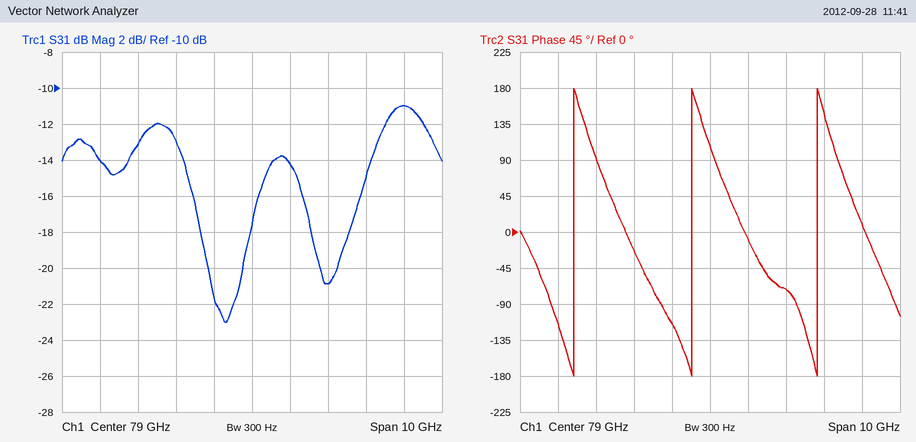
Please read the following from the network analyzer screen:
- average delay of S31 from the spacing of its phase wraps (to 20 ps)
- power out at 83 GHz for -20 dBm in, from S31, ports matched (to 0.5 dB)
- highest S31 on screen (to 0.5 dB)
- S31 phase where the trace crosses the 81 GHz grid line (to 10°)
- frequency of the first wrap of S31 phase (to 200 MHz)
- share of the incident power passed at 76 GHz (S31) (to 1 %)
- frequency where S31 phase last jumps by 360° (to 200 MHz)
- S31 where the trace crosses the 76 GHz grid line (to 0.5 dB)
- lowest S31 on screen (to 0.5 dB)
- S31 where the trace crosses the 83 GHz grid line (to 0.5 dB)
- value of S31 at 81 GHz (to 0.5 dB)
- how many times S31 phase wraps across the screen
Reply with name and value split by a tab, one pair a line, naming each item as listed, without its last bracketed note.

average delay of S31 from the spacing of its phase wraps	320 ps
power out at 83 GHz for -20 dBm in, from S31, ports matched	-31.0 dBm
highest S31 on screen	-11.0 dB
S31 phase where the trace crosses the 81 GHz grid line	-70°
frequency of the first wrap of S31 phase	75.4 GHz
share of the incident power passed at 76 GHz (S31)	5 %
frequency where S31 phase last jumps by 360°	81.8 GHz
S31 where the trace crosses the 76 GHz grid line	-13.0 dB
lowest S31 on screen	-23.0 dB
S31 where the trace crosses the 83 GHz grid line	-11.0 dB
value of S31 at 81 GHz	-21.0 dB
how many times S31 phase wraps across the screen	3
